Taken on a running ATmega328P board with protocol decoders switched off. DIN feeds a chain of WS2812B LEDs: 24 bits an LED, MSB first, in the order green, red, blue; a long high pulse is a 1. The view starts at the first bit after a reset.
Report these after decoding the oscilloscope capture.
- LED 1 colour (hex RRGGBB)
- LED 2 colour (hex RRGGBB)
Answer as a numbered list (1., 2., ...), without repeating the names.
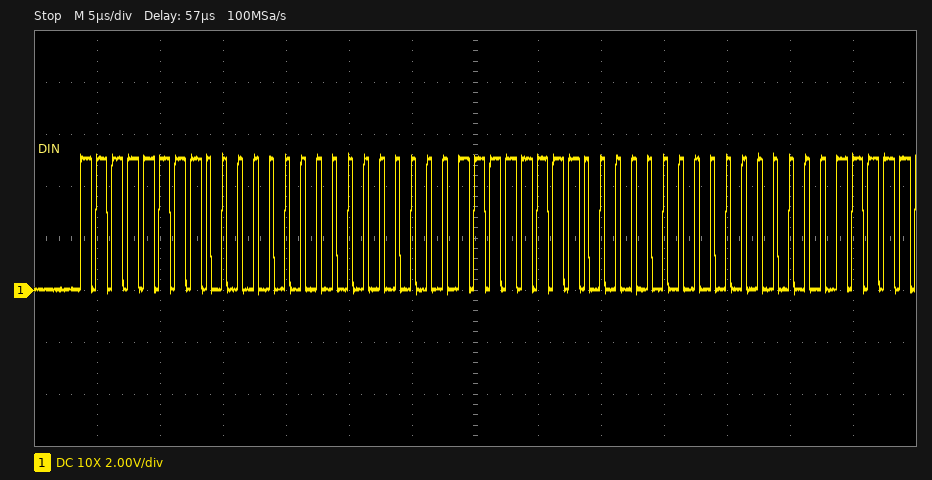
1. #00FF00
2. #00FF00
